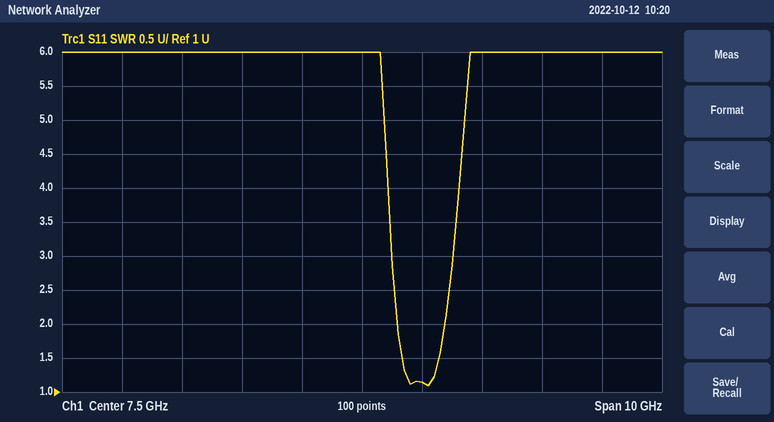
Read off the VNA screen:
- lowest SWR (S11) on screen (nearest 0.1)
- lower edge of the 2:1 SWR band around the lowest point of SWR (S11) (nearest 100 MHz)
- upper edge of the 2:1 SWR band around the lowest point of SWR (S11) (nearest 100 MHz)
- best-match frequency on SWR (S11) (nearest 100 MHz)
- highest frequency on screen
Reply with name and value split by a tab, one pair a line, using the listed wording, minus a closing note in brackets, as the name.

lowest SWR (S11) on screen	1.1
lower edge of the 2:1 SWR band around the lowest point of SWR (S11)	8.1 GHz
upper edge of the 2:1 SWR band around the lowest point of SWR (S11)	8.9 GHz
best-match frequency on SWR (S11)	8.6 GHz
highest frequency on screen	12.5 GHz
